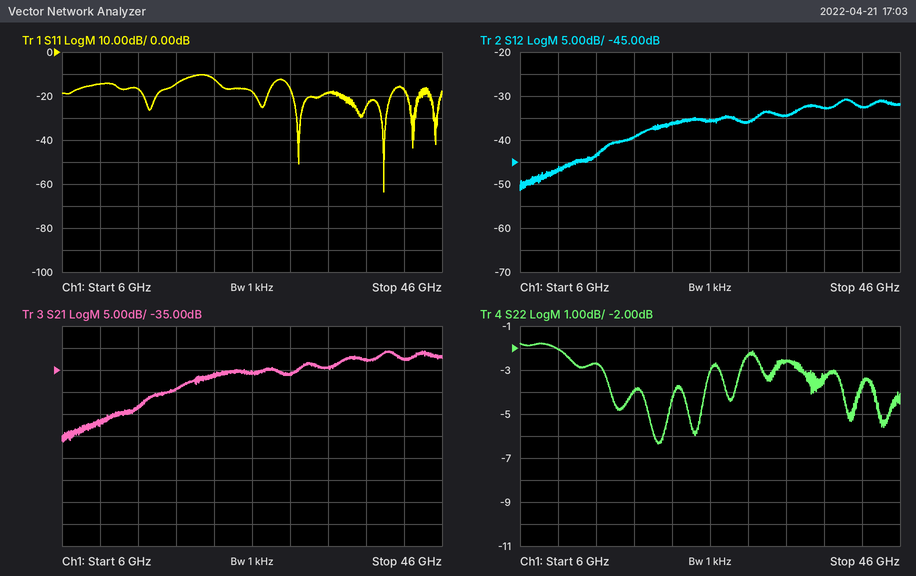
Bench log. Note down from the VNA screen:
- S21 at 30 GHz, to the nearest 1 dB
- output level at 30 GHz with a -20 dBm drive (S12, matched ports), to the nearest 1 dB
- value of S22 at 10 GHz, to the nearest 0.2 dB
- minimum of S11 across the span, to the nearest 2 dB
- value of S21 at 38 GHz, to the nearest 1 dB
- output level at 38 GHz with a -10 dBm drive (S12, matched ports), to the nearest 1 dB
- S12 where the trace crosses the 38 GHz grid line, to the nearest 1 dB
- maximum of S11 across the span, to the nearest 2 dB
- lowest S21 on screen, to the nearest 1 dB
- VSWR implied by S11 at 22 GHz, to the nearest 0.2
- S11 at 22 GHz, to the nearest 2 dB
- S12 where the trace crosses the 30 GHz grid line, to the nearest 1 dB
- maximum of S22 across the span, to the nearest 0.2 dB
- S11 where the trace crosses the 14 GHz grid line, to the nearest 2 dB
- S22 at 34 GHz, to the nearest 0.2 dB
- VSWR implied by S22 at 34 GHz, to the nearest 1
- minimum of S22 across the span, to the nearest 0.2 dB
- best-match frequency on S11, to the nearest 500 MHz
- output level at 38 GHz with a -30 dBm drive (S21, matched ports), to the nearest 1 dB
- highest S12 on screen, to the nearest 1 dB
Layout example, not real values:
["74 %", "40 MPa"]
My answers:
["-36 dB", "-56 dBm", "-2.0 dB", "-64 dB", "-33 dB", "-43 dBm", "-33 dB", "-10 dB", "-51 dB", "1.6", "-12 dB", "-36 dB", "-1.8 dB", "-16 dB", "-2.6 dB", "7", "-6.4 dB", "40.0 GHz", "-63 dBm", "-31 dB"]
